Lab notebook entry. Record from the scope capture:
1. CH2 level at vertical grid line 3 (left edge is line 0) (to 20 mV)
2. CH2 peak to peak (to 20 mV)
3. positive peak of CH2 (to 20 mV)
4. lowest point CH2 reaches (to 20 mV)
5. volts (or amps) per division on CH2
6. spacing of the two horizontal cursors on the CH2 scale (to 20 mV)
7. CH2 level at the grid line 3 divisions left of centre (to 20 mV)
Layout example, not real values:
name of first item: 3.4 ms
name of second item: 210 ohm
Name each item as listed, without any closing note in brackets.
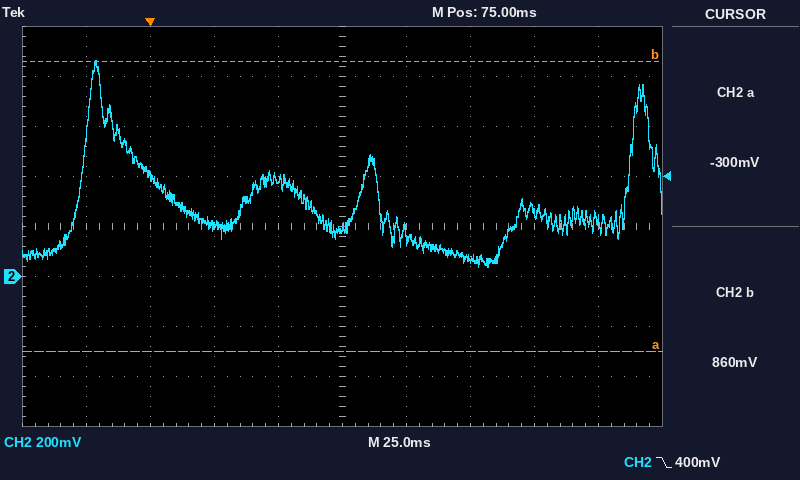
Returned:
CH2 level at vertical grid line 3 (left edge is line 0): 200 mV
CH2 peak to peak: 820 mV
positive peak of CH2: 860 mV
lowest point CH2 reaches: 40 mV
volts (or amps) per division on CH2: 200 mV
spacing of the two horizontal cursors on the CH2 scale: 1.16 V
CH2 level at the grid line 3 divisions left of centre: 400 mV
